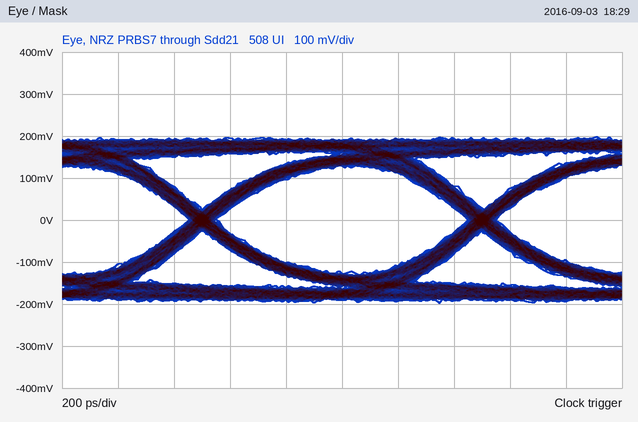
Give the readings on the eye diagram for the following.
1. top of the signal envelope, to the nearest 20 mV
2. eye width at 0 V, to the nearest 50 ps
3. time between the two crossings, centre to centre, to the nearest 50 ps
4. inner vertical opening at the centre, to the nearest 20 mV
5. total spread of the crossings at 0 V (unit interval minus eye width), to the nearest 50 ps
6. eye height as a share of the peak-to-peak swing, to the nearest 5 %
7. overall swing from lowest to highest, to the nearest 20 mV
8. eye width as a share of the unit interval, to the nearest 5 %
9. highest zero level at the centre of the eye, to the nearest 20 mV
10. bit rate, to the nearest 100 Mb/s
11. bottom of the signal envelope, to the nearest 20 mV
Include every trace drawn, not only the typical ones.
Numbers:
200 mV
900 ps
1.00 ns
260 mV
100 ps
65 %
400 mV
90 %
-120 mV
1.0 Gb/s
-200 mV
